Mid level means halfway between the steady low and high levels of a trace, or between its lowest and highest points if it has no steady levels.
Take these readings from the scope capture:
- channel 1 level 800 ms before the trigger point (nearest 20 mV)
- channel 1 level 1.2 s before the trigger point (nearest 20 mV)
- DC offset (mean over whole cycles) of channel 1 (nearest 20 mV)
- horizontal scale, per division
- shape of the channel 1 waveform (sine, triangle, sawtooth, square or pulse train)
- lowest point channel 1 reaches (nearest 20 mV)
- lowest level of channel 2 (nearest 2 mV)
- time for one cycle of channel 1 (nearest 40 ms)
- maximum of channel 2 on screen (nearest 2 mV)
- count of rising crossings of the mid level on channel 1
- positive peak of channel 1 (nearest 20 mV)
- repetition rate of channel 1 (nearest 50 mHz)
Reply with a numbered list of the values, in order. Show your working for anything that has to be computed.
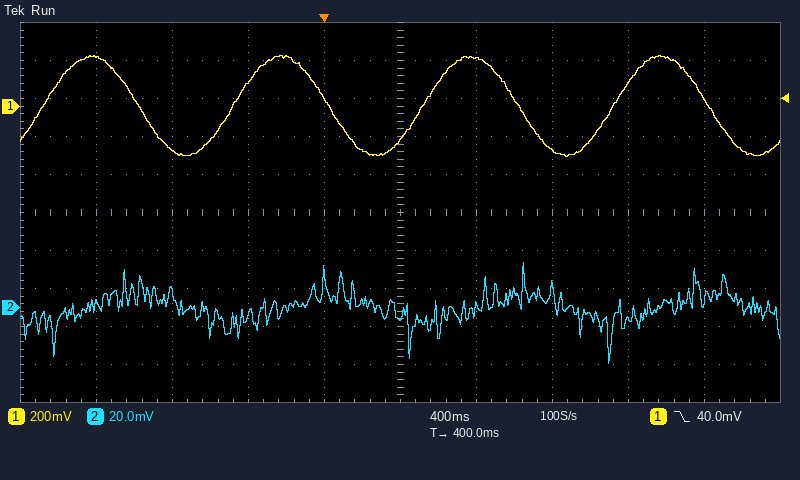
1. -240 mV
2. 260 mV
3. (260 mV + (-260 mV)) / 2 ≈ 0 mV
4. 400 ms
5. sine
6. -260 mV
7. -30 mV
8. 1.00 s
9. 24 mV
10. 4
11. 260 mV
12. 1 / 1.00 s ≈ 1.00 Hz
